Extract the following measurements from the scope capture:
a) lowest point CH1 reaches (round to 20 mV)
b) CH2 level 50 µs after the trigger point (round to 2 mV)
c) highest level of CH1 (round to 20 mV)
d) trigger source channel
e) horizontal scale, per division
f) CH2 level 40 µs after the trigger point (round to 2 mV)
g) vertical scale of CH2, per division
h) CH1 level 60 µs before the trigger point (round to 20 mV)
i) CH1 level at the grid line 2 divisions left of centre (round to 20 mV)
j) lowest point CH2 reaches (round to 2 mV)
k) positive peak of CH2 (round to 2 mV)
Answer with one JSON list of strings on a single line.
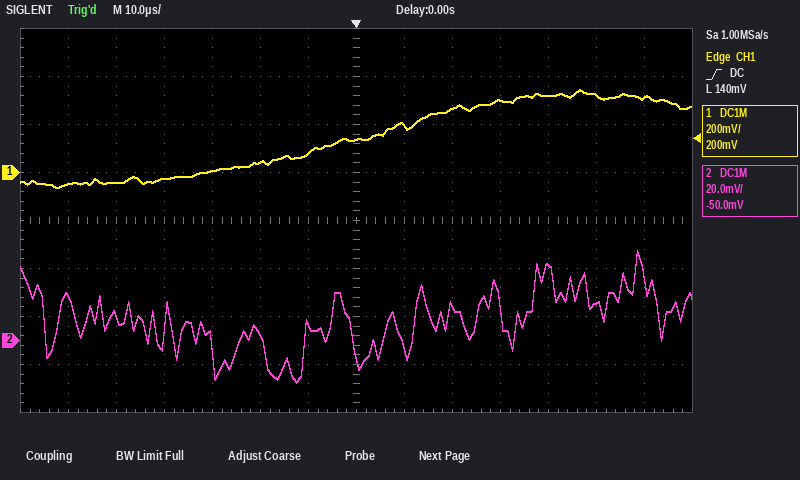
["-60 mV", "16 mV", "340 mV", "CH1", "10 µs", "32 mV", "20 mV", "-40 mV", "40 mV", "-18 mV", "38 mV"]
